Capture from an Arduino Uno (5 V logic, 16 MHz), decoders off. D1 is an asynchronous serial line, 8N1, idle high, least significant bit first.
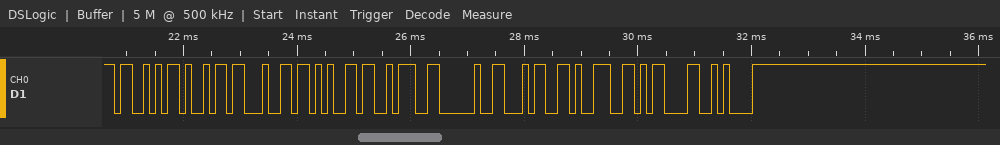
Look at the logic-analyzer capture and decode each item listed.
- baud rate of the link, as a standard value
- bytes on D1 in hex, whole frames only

9600 baud
0x53 0x69 0x64 0x65 0x3A 0x20 0x34 0x39 0x0D 0x0A
